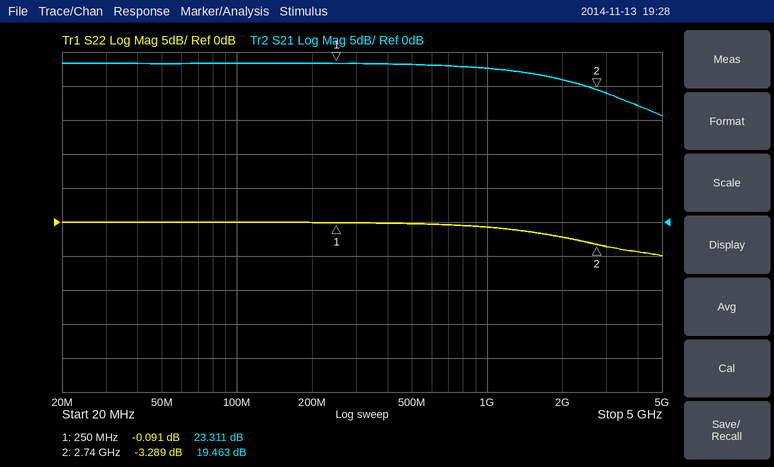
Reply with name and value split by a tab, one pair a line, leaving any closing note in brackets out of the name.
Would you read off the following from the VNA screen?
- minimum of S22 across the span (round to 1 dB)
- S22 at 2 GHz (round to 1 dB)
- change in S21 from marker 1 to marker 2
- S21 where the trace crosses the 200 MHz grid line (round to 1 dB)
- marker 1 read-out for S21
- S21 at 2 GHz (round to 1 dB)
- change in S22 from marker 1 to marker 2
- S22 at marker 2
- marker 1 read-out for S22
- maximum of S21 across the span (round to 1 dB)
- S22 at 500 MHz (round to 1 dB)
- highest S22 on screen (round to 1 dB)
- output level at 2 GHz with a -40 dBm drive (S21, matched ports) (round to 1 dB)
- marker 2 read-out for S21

minimum of S22 across the span	-5 dB
S22 at 2 GHz	-2 dB
change in S21 from marker 1 to marker 2	-3.848 dB
S21 where the trace crosses the 200 MHz grid line	23 dB
marker 1 read-out for S21	23.311 dB
S21 at 2 GHz	21 dB
change in S22 from marker 1 to marker 2	-3.198 dB
S22 at marker 2	-3.289 dB
marker 1 read-out for S22	-0.091 dB
maximum of S21 across the span	23 dB
S22 at 500 MHz	0 dB
highest S22 on screen	0 dB
output level at 2 GHz with a -40 dBm drive (S21, matched ports)	-19 dBm
marker 2 read-out for S21	19.463 dB
